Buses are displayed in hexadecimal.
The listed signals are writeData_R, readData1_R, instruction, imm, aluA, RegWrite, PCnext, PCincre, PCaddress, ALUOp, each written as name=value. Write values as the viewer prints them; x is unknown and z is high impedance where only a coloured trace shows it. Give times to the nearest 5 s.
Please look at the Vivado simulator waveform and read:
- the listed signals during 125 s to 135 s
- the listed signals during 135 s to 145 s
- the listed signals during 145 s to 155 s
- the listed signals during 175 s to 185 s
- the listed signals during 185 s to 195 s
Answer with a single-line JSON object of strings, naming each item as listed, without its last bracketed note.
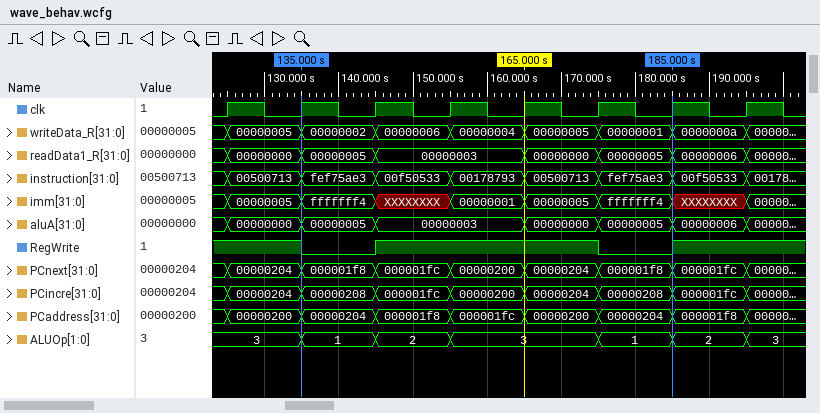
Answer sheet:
{"the listed signals during 125 s to 135 s": "writeData_R=00000005, readData1_R=00000000, instruction=00500713, imm=00000005, aluA=00000000, RegWrite=1, PCnext=00000204, PCincre=00000204, PCaddress=00000200, ALUOp=3", "the listed signals during 135 s to 145 s": "writeData_R=00000002, readData1_R=00000005, instruction=fef75ae3, imm=fffffff4, aluA=00000005, RegWrite=0, PCnext=000001f8, PCincre=00000208, PCaddress=00000204, ALUOp=1", "the listed signals during 145 s to 155 s": "writeData_R=00000006, readData1_R=00000003, instruction=00f50533, imm=XXXXXXXX, aluA=00000003, RegWrite=1, PCnext=000001fc, PCincre=000001fc, PCaddress=000001f8, ALUOp=2", "the listed signals during 175 s to 185 s": "writeData_R=00000001, readData1_R=00000005, instruction=fef75ae3, imm=fffffff4, aluA=00000005, RegWrite=0, PCnext=000001f8, PCincre=00000208, PCaddress=00000204, ALUOp=1", "the listed signals during 185 s to 195 s": "writeData_R=0000000a, readData1_R=00000006, instruction=00f50533, imm=XXXXXXXX, aluA=00000006, RegWrite=1, PCnext=000001fc, PCincre=000001fc, PCaddress=000001f8, ALUOp=2"}
